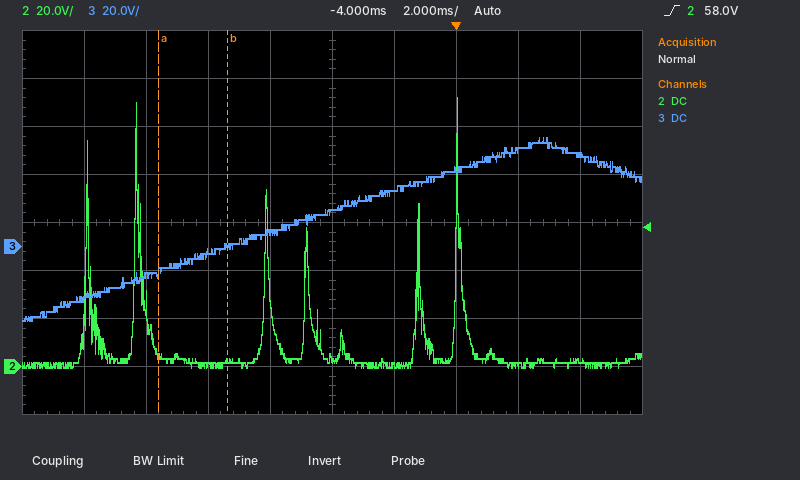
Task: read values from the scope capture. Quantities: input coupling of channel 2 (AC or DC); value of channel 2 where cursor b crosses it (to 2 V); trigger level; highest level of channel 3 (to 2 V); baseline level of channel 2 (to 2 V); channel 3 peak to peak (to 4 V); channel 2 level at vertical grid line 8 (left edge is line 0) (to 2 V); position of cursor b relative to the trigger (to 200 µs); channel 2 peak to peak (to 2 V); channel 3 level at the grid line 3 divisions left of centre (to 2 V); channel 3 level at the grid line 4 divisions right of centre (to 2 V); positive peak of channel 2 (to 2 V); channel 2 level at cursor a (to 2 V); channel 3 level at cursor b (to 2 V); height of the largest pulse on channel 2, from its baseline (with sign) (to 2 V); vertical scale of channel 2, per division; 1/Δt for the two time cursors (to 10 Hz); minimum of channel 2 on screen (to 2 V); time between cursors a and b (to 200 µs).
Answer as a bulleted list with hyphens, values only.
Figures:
- DC
- 2 V
- 58.0 V
- 46 V
- 2 V
- 76 V
- 0 V
- -7.4 ms
- 112 V
- -12 V
- 38 V
- 112 V
- 6 V
- 0 V
- +110 V
- 20 V
- 450 Hz
- 0 V
- 2.2 ms
